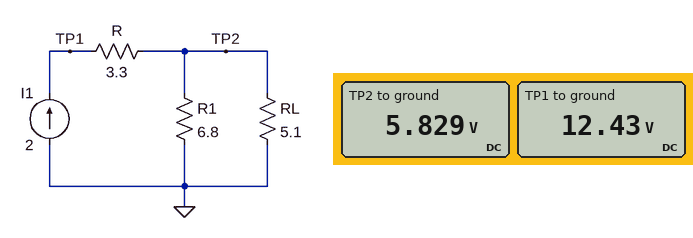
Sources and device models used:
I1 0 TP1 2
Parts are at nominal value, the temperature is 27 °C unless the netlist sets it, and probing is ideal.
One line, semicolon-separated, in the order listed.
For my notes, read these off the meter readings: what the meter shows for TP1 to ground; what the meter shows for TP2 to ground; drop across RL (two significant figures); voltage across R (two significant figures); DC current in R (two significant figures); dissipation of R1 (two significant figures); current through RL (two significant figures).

12.43 V; 5.829 V; 5.8 V; 6.6 V; 2.0 A; 5.0 W; 1.1 A
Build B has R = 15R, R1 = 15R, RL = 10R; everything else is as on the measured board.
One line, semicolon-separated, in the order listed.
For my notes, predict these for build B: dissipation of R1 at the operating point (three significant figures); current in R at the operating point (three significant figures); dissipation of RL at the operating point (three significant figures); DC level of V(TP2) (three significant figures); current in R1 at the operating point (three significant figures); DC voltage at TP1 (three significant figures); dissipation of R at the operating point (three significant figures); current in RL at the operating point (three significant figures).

9.60 W; 2.00 A; 14.4 W; 12.0 V; 800 mA; 42.0 V; 60.0 W; 1.20 A
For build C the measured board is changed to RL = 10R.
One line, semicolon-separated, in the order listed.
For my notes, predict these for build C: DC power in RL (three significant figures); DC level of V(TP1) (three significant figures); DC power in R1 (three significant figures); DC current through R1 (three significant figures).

6.55 W; 14.7 V; 9.64 W; 1.19 A
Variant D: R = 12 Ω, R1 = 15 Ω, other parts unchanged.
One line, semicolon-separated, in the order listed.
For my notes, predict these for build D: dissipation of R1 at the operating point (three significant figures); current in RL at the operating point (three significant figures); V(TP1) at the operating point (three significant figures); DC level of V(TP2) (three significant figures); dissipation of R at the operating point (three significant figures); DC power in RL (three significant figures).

3.86 W; 1.49 A; 31.6 V; 7.61 V; 48.0 W; 11.4 W
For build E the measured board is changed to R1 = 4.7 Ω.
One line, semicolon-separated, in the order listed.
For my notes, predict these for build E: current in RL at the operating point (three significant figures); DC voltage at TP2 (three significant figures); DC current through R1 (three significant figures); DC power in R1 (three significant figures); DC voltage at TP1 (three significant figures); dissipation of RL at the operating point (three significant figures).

959 mA; 4.89 V; 1.04 A; 5.09 W; 11.5 V; 4.69 W
